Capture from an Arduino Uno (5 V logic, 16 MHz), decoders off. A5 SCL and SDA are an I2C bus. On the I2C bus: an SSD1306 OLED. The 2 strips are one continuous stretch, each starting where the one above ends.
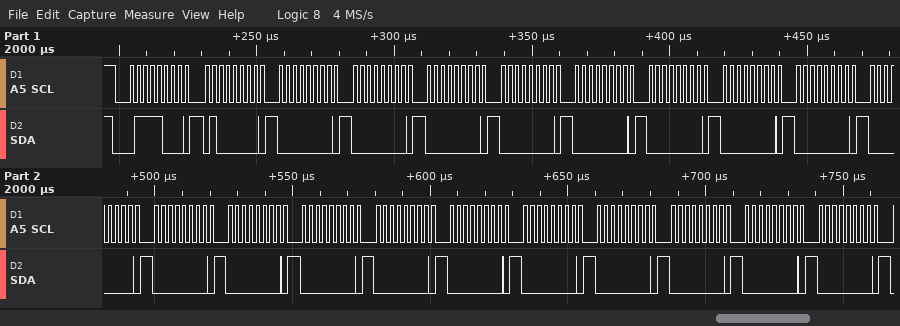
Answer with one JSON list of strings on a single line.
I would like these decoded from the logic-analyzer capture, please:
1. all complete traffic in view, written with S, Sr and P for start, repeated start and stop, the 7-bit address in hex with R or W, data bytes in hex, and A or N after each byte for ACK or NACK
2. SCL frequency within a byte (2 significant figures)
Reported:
["S 3CW A 40 A 00 A 00 A 00 A 00 A 00 A 00 A 00 A 00 A 00 A 00 A 00 A 00 A 00 A 00 A 00 A 00 A 00 A 00 A 00 A", "400 kHz"]
